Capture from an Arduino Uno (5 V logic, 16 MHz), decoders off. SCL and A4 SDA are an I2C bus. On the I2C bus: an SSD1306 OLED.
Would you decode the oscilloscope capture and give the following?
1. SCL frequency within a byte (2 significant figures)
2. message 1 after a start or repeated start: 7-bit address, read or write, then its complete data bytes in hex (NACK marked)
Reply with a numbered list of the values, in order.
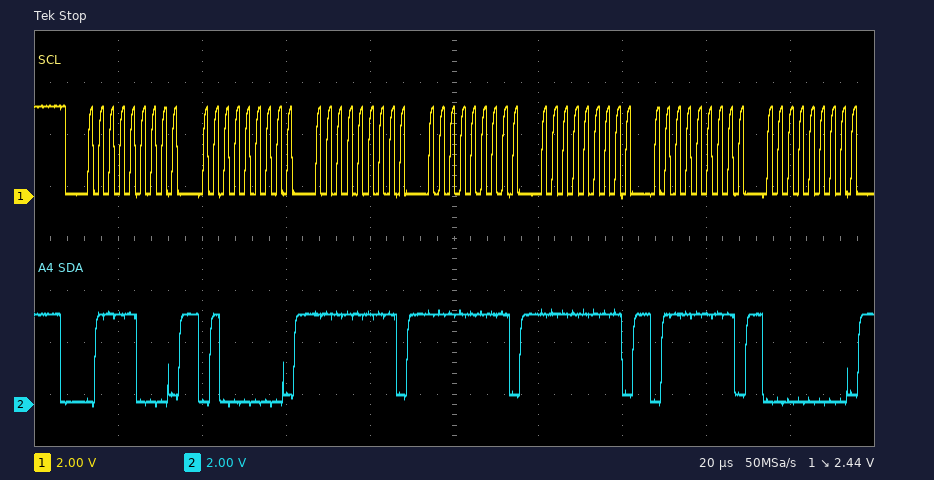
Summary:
1. 400 kHz
2. 0x3C write: 40 FF FF FF 7F 00
